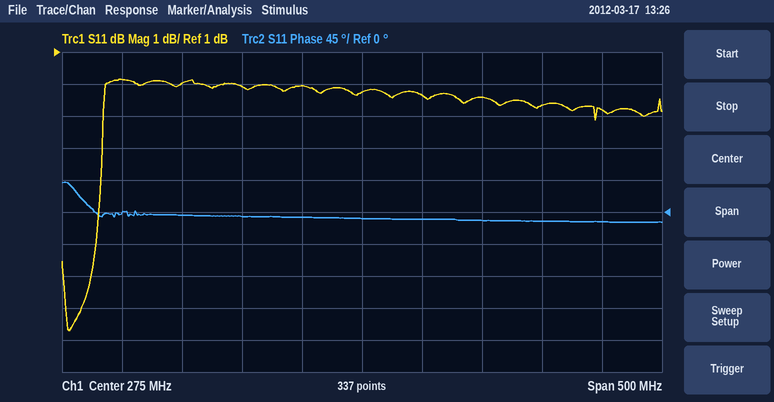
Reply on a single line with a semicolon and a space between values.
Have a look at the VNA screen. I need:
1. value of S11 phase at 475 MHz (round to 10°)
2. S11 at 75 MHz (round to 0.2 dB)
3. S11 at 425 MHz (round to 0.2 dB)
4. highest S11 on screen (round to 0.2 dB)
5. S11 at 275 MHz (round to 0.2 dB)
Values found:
-10°; 0.2 dB; -0.6 dB; 0.2 dB; -0.2 dB
